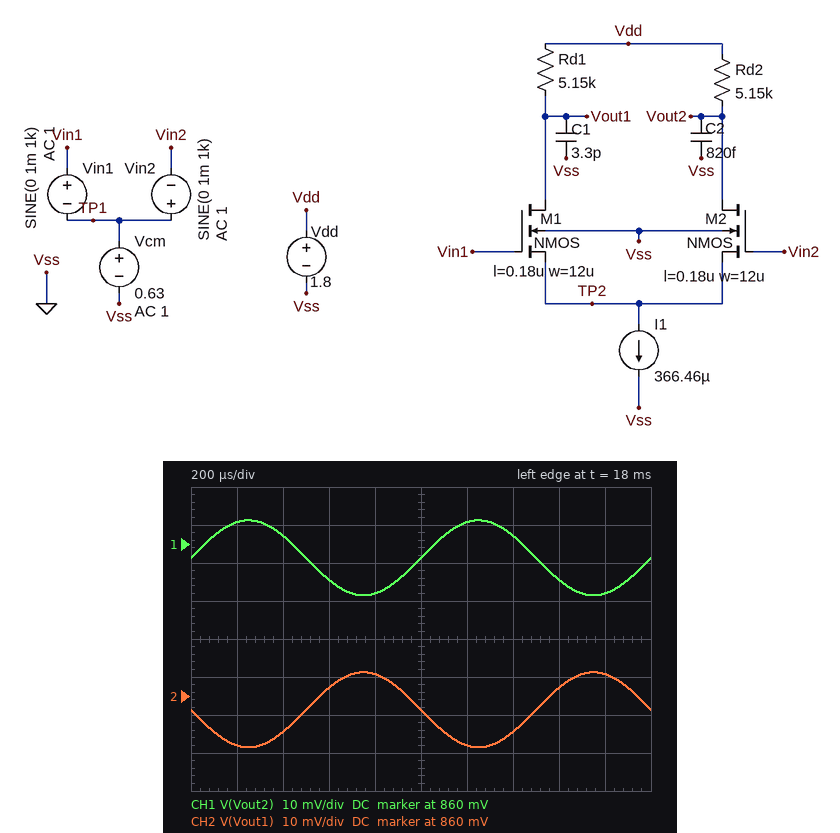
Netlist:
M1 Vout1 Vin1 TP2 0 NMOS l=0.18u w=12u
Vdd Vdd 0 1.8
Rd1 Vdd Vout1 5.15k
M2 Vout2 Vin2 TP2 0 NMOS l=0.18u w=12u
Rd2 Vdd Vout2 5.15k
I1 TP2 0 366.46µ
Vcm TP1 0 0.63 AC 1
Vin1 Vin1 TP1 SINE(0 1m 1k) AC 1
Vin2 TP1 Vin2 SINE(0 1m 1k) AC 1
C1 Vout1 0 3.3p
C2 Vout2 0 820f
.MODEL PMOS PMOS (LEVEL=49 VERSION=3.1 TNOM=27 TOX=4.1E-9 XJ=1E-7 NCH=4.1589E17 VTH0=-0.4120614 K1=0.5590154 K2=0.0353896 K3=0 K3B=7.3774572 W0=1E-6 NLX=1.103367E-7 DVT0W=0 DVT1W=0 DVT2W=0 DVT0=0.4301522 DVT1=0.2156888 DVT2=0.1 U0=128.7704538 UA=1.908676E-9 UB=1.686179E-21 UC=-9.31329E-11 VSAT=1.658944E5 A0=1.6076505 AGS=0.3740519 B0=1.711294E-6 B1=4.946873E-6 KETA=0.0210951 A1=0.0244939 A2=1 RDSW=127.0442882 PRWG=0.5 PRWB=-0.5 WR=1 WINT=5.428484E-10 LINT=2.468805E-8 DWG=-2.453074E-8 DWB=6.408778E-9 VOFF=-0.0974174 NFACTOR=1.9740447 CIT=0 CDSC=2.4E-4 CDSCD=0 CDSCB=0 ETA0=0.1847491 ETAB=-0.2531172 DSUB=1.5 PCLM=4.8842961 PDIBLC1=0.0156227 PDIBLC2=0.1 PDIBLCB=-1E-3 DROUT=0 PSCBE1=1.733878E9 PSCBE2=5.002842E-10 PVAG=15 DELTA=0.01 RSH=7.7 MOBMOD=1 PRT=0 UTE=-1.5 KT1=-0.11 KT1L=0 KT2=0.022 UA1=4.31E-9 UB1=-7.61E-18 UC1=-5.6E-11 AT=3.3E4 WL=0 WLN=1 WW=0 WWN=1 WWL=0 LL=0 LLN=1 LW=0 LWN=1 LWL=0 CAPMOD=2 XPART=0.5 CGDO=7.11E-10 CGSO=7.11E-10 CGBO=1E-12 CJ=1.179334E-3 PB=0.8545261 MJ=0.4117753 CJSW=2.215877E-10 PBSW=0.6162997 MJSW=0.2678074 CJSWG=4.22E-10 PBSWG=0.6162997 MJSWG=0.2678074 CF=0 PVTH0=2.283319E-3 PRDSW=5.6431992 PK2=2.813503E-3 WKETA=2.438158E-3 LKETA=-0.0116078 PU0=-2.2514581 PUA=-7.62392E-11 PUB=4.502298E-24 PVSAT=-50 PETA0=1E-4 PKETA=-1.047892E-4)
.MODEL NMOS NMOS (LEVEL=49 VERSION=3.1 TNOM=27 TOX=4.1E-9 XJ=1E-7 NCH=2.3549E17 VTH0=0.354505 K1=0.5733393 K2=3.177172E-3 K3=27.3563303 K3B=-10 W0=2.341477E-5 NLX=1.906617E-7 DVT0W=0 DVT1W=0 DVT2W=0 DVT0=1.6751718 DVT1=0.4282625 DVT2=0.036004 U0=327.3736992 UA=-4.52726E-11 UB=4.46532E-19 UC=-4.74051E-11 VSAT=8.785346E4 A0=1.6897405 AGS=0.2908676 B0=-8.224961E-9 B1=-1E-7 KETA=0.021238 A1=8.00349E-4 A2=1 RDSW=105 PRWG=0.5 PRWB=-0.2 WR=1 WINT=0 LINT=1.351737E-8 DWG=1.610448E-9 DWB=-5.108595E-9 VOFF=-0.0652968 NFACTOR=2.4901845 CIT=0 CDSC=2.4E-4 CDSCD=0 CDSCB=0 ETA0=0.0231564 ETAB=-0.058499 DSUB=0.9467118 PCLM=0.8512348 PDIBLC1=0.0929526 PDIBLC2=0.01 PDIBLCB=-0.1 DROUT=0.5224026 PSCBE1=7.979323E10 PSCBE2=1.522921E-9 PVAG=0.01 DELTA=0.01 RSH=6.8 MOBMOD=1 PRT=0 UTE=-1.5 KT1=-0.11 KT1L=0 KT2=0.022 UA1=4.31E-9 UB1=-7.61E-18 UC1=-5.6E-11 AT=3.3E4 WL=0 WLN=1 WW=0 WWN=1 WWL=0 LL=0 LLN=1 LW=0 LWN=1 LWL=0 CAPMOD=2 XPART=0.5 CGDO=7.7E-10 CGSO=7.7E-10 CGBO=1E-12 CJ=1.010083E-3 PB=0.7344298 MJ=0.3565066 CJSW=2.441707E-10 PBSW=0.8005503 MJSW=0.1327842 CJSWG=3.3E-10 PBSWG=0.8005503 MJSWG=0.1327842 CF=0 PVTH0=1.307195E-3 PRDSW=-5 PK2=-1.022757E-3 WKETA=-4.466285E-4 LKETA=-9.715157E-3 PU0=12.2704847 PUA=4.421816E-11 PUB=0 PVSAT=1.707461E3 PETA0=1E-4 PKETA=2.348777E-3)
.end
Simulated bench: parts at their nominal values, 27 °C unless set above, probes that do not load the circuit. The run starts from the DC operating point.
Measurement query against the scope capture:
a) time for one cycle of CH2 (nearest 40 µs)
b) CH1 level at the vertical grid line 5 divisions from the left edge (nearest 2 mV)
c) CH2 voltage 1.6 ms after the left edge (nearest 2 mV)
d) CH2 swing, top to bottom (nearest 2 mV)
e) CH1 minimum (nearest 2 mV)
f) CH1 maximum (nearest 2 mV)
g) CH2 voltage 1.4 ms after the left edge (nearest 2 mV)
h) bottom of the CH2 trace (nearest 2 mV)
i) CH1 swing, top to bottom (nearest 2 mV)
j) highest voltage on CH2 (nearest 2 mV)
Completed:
1.00 ms
856 mV
862 mV
20 mV
846 mV
866 mV
850 mV
846 mV
20 mV
866 mV
